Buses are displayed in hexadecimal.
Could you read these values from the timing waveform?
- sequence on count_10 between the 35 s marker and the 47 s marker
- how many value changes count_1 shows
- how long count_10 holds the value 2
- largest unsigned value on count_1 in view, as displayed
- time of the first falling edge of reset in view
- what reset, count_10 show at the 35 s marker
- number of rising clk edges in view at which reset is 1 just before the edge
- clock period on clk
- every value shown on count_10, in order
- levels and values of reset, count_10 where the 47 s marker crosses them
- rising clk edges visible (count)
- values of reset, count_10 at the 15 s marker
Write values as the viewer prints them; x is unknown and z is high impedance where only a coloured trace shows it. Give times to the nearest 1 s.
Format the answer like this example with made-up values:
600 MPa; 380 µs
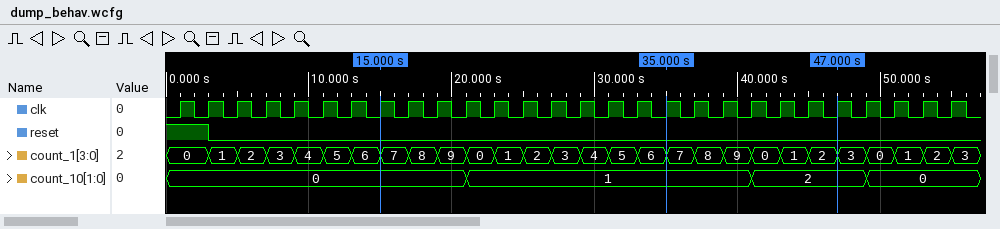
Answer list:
1, 2; 27; 8 s; 9; 3 s; reset=0, count_10=1; 2; 2 s; 0, 1, 2, 0; reset=0, count_10=2; 28; reset=0, count_10=0
